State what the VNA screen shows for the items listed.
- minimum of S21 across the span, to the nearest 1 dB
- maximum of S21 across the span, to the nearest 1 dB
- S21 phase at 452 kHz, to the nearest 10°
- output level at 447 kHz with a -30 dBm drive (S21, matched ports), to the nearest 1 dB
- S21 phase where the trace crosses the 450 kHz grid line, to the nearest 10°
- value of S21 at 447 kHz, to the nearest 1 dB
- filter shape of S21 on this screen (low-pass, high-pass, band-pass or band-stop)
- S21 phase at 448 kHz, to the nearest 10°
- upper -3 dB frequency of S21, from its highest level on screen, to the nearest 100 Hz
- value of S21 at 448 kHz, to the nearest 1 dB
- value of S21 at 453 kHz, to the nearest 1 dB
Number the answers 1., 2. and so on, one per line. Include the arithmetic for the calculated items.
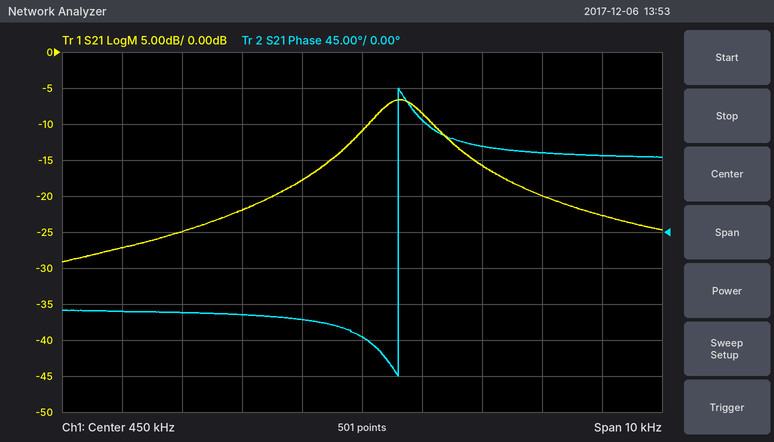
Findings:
1. -29 dB
2. -7 dB
3. 110°
4. -30 dBm + (-25 dB) = -55 dBm
5. -130°
6. -25 dB
7. band-pass
8. -100°
9. 451.1 kHz
10. -22 dB
11. -20 dB
